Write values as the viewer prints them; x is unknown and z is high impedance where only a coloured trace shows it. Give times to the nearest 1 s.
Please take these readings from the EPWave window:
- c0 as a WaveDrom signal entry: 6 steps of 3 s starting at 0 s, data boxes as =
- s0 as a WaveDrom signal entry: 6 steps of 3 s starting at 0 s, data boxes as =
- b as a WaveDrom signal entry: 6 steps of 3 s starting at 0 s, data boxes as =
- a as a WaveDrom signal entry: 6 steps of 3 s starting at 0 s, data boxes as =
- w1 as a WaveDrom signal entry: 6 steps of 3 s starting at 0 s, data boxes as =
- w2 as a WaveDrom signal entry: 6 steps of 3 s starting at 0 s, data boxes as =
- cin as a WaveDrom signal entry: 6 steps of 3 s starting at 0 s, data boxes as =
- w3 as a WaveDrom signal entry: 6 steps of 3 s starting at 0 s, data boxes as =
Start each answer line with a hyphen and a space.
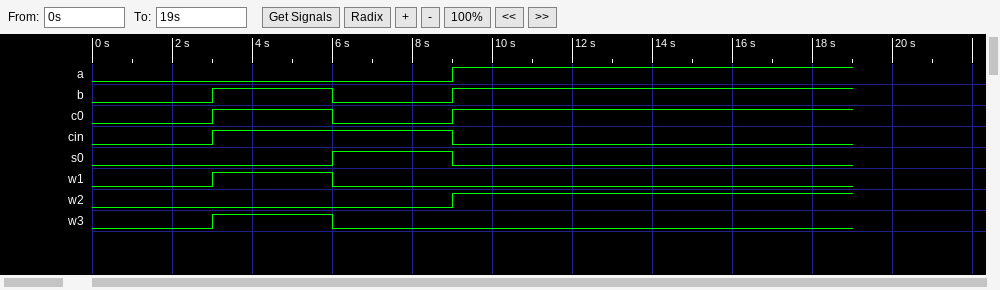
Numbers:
- {name: 'c0', wave: '0101..'}
- {name: 's0', wave: '0.10..'}
- {name: 'b', wave: '0101..'}
- {name: 'a', wave: '0..1..'}
- {name: 'w1', wave: '010...'}
- {name: 'w2', wave: '0..1..'}
- {name: 'cin', wave: '01.0..'}
- {name: 'w3', wave: '010...'}
